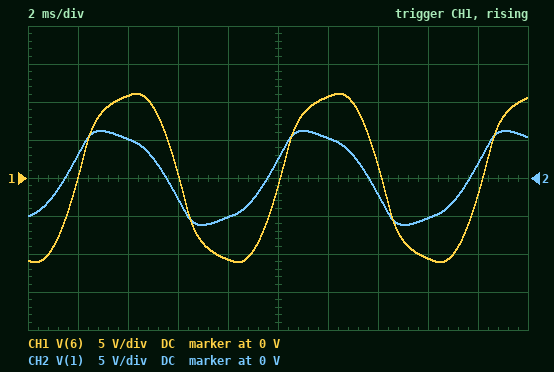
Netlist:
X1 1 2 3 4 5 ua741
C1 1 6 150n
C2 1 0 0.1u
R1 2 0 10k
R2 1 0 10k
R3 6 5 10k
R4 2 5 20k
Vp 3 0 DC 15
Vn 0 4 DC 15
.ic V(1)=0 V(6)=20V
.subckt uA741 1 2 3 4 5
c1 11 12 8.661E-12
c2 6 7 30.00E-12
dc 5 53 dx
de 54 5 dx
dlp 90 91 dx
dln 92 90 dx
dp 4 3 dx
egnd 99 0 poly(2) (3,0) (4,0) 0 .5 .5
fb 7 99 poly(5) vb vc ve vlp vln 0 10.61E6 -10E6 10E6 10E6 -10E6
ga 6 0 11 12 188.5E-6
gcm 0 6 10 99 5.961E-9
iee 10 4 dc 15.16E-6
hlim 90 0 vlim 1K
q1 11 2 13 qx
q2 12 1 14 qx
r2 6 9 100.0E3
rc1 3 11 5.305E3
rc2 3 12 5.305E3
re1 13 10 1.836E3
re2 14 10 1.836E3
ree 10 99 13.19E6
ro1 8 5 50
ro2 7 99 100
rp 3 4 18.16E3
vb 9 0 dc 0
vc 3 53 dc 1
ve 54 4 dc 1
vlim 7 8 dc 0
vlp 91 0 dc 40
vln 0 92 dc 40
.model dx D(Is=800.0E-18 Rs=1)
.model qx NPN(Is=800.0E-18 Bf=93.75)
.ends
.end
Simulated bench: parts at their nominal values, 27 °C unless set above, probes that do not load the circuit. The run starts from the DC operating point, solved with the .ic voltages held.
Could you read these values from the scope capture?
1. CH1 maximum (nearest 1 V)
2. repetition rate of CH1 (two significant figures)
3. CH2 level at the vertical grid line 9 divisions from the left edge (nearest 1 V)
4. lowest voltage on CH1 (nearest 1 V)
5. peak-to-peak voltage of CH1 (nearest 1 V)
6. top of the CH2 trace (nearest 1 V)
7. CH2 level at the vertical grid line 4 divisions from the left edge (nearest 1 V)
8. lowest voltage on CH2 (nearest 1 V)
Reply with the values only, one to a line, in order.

11 V
120 Hz
2 V
-11 V
22 V
6 V
-5 V
-6 V
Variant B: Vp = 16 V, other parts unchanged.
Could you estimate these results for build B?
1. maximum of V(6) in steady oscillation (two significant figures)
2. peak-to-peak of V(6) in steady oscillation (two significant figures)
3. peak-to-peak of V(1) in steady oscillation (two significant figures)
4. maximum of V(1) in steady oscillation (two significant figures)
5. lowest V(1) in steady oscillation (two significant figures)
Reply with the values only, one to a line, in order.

12 V
23 V
13 V
6.5 V
-6.3 V
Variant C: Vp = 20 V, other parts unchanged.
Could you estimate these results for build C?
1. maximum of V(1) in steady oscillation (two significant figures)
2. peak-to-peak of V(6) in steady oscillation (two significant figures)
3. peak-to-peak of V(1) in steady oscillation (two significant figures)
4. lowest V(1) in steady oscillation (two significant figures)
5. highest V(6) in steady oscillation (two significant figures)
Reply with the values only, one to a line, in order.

7.6 V
26 V
14 V
-6.8 V
15 V
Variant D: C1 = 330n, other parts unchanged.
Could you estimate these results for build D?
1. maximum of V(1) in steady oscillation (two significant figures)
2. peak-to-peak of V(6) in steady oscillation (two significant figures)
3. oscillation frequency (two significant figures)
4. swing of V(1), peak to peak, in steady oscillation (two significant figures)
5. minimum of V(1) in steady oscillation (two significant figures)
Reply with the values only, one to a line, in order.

7.7 V
21 V
70 Hz
15 V
-7.7 V
